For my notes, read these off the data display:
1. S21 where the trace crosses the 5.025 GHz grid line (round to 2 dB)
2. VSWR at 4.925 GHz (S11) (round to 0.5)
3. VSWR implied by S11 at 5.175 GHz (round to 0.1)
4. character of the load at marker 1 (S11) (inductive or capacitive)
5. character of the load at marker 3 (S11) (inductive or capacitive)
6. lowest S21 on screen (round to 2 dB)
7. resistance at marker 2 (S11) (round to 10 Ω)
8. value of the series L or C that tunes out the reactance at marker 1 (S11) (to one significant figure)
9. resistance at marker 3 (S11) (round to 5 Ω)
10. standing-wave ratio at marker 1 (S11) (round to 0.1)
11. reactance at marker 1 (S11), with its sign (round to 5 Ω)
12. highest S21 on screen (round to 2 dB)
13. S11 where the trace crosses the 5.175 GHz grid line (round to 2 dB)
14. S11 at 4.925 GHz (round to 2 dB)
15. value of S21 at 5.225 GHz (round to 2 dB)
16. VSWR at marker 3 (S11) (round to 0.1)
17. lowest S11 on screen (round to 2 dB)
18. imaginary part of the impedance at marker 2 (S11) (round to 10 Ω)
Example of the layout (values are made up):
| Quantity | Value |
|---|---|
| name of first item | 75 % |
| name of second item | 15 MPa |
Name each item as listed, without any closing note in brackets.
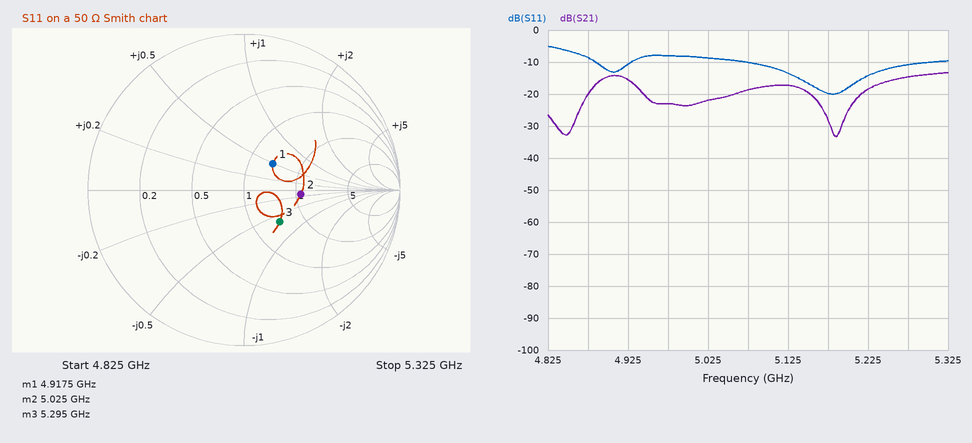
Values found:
| Quantity | Value |
|---|---|
| S21 where the trace crosses the 5.025 GHz grid line | -22 dB |
| VSWR at 4.925 GHz (S11) | 2.0 |
| VSWR implied by S11 at 5.175 GHz | 1.2 |
| character of the load at marker 1 (S11) | inductive |
| character of the load at marker 3 (S11) | capacitive |
| lowest S21 on screen | -34 dB |
| resistance at marker 2 (S11) | 110 Ω |
| value of the series L or C that tunes out the reactance at marker 1 (S11) | 1 pF |
| resistance at marker 3 (S11) | 70 Ω |
| standing-wave ratio at marker 1 (S11) | 1.7 |
| reactance at marker 1 (S11), with its sign | +25 Ω |
| highest S21 on screen | -14 dB |
| S11 where the trace crosses the 5.175 GHz grid line | -20 dB |
| S11 at 4.925 GHz | -10 dB |
| value of S21 at 5.225 GHz | -18 dB |
| VSWR at marker 3 (S11) | 1.9 |
| lowest S11 on screen | -20 dB |
| imaginary part of the impedance at marker 2 (S11) | -10 Ω |
